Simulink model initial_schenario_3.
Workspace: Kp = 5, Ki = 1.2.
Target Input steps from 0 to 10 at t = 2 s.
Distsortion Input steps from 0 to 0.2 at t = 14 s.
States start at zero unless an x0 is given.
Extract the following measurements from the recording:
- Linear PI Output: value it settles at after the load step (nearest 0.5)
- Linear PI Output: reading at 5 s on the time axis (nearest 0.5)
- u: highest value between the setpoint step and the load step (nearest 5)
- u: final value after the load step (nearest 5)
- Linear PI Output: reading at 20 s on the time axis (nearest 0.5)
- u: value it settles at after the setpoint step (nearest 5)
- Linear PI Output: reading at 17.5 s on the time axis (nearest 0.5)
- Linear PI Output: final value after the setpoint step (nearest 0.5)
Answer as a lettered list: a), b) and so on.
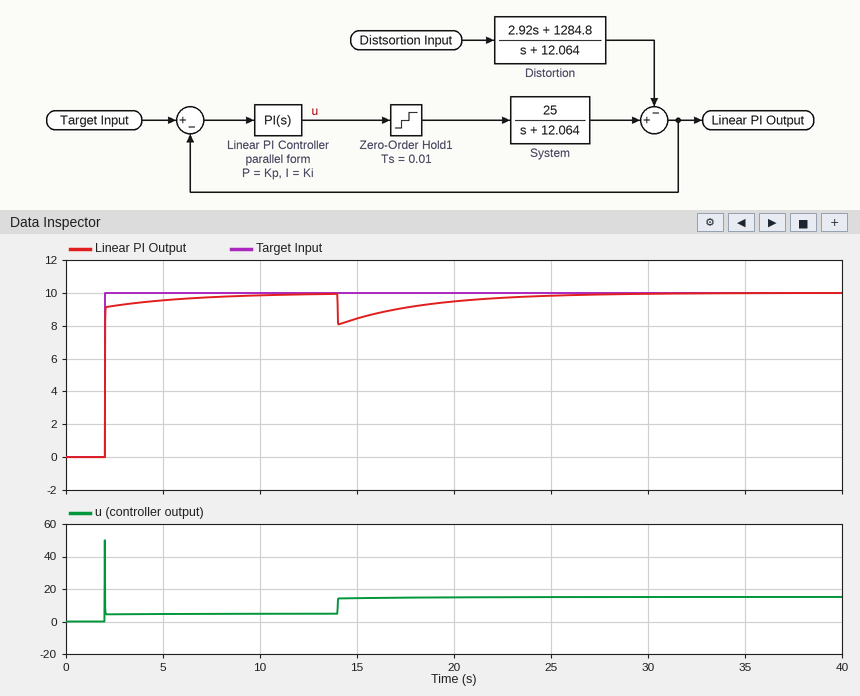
a) 10.0
b) 9.5
c) 50
d) 15
e) 9.5
f) 5
g) 9.0
h) 10.0
